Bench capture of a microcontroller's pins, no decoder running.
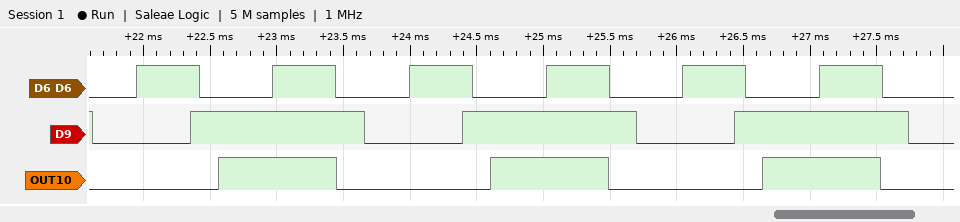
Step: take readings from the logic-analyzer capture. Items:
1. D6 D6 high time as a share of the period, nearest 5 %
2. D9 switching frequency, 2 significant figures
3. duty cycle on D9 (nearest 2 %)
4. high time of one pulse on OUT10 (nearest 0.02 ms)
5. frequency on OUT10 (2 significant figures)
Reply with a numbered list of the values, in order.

1. 45 %
2. 490 Hz
3. 64 %
4. 0.88 ms
5. 490 Hz
